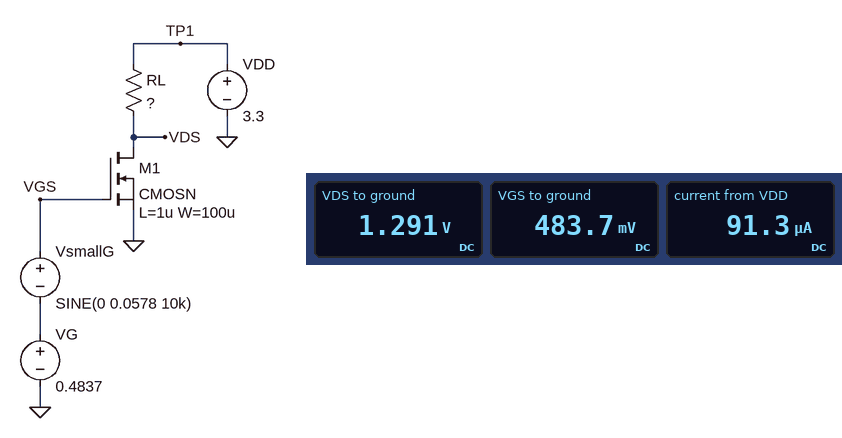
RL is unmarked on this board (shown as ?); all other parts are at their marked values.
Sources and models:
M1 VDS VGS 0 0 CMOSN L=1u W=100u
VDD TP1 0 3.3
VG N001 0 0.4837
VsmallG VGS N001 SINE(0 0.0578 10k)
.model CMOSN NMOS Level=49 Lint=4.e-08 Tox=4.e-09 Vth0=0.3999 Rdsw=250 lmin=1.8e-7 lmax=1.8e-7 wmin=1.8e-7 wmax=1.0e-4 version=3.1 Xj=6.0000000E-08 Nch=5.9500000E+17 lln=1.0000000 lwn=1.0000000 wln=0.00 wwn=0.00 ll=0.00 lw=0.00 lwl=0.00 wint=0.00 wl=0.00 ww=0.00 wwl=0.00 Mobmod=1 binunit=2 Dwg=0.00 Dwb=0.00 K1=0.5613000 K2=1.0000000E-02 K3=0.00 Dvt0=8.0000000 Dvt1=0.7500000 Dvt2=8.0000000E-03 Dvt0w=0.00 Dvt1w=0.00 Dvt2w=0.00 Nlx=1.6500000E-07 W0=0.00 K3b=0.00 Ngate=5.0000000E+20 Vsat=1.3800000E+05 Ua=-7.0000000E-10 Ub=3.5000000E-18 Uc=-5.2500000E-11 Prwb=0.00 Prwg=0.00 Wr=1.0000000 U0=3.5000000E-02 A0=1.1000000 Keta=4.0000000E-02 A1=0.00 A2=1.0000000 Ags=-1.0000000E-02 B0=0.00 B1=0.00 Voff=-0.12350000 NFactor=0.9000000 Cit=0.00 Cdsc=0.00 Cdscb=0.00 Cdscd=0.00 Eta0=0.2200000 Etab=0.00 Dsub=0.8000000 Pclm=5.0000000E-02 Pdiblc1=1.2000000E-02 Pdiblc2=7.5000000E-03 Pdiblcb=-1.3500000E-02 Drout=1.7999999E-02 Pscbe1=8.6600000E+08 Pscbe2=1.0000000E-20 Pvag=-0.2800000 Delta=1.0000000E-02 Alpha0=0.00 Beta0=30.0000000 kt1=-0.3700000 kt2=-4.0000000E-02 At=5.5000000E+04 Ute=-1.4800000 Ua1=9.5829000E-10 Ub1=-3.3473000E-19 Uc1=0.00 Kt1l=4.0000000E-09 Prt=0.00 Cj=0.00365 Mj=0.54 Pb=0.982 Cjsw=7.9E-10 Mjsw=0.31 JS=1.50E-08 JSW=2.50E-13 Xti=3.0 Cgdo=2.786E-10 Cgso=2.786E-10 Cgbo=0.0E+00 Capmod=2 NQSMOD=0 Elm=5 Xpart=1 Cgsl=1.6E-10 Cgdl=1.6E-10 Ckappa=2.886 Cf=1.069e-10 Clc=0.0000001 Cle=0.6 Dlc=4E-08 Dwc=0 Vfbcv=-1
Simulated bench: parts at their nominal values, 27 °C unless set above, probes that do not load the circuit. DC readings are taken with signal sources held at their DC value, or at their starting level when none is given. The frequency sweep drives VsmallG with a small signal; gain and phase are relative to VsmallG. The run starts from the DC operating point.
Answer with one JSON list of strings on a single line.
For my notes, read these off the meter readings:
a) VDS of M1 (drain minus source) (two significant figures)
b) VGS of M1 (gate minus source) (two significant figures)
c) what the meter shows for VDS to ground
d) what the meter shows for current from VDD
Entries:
["1.3 V", "480 mV", "1.291 V", "91.3 µA"]
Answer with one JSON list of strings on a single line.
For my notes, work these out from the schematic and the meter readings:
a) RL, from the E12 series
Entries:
["22 kΩ"]
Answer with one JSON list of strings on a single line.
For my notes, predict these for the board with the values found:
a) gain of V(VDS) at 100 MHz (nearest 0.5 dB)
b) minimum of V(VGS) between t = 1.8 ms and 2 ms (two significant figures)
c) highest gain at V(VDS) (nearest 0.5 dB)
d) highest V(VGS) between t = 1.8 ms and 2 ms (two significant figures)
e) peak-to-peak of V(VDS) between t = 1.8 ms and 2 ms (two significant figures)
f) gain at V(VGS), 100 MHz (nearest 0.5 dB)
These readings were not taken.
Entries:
["24.5 dB", "430 mV", "28.5 dB", "540 mV", "2.4 V", "0 dB"]
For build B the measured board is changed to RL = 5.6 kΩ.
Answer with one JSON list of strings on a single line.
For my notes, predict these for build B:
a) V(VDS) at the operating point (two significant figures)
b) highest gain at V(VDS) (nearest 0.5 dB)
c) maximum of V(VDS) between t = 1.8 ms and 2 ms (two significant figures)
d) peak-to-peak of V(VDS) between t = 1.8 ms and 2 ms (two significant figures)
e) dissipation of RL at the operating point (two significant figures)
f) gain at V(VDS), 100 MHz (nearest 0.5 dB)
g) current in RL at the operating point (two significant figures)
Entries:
["2.7 V", "19.5 dB", "3.1 V", "1.1 V", "63 µW", "19.0 dB", "110 µA"]
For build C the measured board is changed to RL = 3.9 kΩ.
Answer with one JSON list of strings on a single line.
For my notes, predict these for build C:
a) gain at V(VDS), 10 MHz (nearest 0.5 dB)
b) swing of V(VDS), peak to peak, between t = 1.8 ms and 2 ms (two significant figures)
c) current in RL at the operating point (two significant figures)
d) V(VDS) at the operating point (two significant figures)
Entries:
["16.5 dB", "780 mV", "110 µA", "2.9 V"]
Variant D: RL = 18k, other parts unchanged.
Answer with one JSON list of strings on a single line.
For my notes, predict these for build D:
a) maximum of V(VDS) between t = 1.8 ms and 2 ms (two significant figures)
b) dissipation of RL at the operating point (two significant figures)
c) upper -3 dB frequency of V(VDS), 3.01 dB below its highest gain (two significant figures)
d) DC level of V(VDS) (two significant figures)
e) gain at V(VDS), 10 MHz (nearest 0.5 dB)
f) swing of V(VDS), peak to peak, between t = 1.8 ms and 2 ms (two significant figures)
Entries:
["2.6 V", "160 µW", "98 MHz", "1.6 V", "27.5 dB", "2.5 V"]
